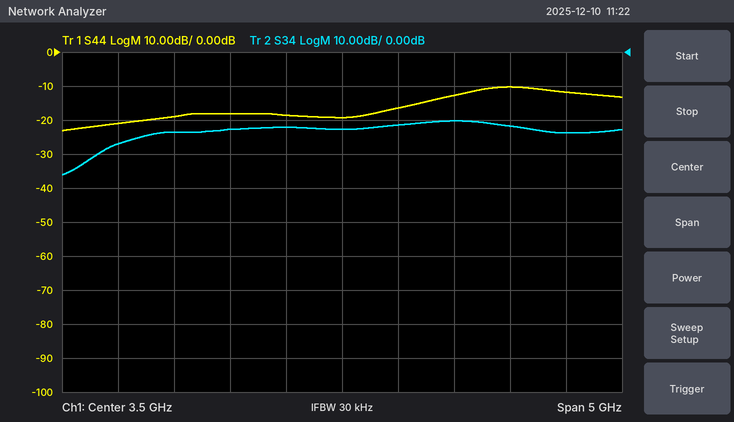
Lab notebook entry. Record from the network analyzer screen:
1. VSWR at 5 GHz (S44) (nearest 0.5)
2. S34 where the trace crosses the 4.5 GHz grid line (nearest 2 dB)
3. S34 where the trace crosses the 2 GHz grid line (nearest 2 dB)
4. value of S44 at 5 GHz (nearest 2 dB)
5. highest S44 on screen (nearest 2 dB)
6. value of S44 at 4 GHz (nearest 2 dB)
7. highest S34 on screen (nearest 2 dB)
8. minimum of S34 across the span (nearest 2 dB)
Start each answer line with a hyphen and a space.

- 2.0
- -20 dB
- -24 dB
- -10 dB
- -10 dB
- -16 dB
- -20 dB
- -36 dB
